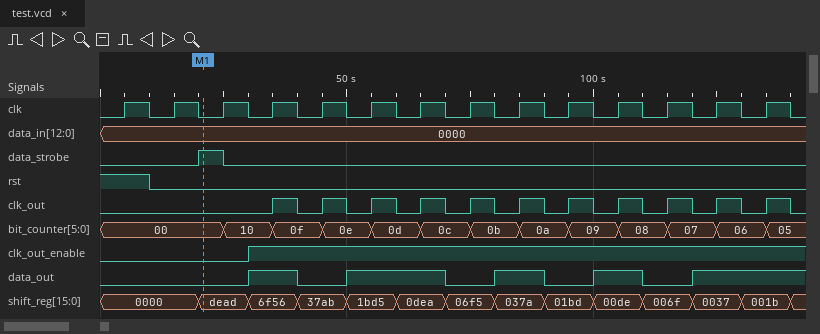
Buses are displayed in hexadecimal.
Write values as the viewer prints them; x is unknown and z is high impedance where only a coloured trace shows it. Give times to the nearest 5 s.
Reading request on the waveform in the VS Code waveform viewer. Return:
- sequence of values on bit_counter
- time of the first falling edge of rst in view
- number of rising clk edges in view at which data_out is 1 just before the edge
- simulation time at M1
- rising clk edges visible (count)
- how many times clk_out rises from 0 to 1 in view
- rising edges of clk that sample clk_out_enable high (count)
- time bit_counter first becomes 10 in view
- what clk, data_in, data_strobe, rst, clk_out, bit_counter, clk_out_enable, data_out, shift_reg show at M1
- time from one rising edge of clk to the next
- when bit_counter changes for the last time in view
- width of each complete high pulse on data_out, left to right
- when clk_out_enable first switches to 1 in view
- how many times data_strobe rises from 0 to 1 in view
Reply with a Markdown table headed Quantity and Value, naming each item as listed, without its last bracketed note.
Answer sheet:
| Quantity | Value |
|---|---|
| sequence of values on bit_counter | 00, 10, 0f, 0e, 0d, 0c, 0b, 0a, 09, 08, 07, 06, 05 |
| time of the first falling edge of rst in view | 10 s |
| number of rising clk edges in view at which data_out is 1 just before the edge | 7 |
| simulation time at M1 | 20 s |
| rising clk edges visible | 14 |
| how many times clk_out rises from 0 to 1 in view | 11 |
| rising edges of clk that sample clk_out_enable high | 11 |
| time bit_counter first becomes 10 in view | 25 s |
| what clk, data_in, data_strobe, rst, clk_out, bit_counter, clk_out_enable, data_out, shift_reg show at M1 | clk=0, data_in=0000, data_strobe=1, rst=0, clk_out=0, bit_counter=00, clk_out_enable=0, data_out=0, shift_reg=dead |
| time from one rising edge of clk to the next | 10 s |
| when bit_counter changes for the last time in view | 135 s |
| width of each complete high pulse on data_out, left to right | 10 s, 20 s, 10 s, 10 s |
| when clk_out_enable first switches to 1 in view | 30 s |
| how many times data_strobe rises from 0 to 1 in view | 1 |
